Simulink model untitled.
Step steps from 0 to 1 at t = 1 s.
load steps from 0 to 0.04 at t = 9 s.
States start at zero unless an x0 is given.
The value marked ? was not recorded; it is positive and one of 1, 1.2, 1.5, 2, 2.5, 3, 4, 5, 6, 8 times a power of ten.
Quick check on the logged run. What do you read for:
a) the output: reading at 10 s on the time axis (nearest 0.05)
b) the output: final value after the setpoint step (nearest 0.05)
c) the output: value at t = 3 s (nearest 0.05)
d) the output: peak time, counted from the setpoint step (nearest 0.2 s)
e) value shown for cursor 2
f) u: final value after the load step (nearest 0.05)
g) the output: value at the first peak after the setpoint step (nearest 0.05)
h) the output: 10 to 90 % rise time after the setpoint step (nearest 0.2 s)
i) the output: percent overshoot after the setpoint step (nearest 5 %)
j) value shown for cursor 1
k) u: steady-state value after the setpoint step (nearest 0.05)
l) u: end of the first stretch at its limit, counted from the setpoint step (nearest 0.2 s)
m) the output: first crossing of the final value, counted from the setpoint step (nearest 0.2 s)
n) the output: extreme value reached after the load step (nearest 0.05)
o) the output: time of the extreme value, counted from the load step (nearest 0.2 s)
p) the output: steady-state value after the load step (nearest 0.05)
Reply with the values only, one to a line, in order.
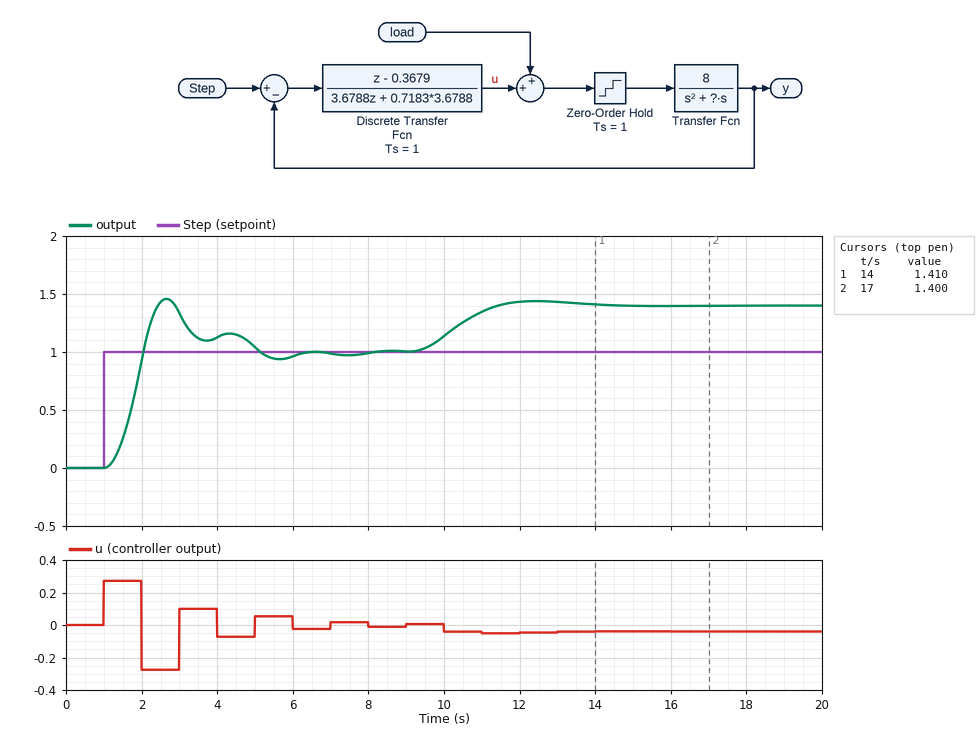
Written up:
1.15
1.00
1.35
1.6 s
1.400
-0.05
1.45
0.6 s
45 %
1.410
0.00
1.0 s
1.0 s
1.45
3.4 s
1.40
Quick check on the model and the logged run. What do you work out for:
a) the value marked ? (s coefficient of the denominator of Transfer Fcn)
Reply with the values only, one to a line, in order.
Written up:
0.5
